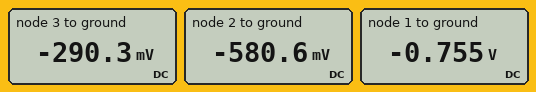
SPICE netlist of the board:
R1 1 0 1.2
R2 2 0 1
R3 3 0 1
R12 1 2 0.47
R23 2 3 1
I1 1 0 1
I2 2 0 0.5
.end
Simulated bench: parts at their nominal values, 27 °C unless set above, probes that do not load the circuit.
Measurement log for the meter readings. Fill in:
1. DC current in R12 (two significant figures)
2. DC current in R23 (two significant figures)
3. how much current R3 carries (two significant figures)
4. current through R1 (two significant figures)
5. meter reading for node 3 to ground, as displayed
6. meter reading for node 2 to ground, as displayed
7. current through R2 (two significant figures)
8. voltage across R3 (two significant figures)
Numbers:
370 mA
290 mA
290 mA
630 mA
-290.3 mV
-580.6 mV
580 mA
290 mV
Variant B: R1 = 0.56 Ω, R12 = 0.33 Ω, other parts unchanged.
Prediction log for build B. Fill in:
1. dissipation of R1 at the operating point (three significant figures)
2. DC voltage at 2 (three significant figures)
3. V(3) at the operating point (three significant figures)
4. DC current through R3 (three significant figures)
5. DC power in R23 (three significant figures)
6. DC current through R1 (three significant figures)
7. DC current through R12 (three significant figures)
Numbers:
409 mW
-430 mV
-215 mV
215 mA
46.3 mW
854 mA
146 mA
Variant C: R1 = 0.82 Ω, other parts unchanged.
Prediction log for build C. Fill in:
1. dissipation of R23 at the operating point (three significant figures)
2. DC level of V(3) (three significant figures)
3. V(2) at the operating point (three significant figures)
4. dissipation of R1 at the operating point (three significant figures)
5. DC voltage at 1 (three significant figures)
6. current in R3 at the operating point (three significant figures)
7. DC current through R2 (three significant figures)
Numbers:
62.3 mW
-250 mV
-499 mV
463 mW
-616 mV
250 mA
499 mA
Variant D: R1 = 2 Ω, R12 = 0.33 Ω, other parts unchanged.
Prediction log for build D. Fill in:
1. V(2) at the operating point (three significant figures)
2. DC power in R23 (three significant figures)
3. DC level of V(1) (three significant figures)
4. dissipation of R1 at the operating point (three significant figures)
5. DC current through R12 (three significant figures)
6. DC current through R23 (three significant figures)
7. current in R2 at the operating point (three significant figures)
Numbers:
-704 mV
124 mW
-888 mV
394 mW
556 mA
352 mA
704 mA
